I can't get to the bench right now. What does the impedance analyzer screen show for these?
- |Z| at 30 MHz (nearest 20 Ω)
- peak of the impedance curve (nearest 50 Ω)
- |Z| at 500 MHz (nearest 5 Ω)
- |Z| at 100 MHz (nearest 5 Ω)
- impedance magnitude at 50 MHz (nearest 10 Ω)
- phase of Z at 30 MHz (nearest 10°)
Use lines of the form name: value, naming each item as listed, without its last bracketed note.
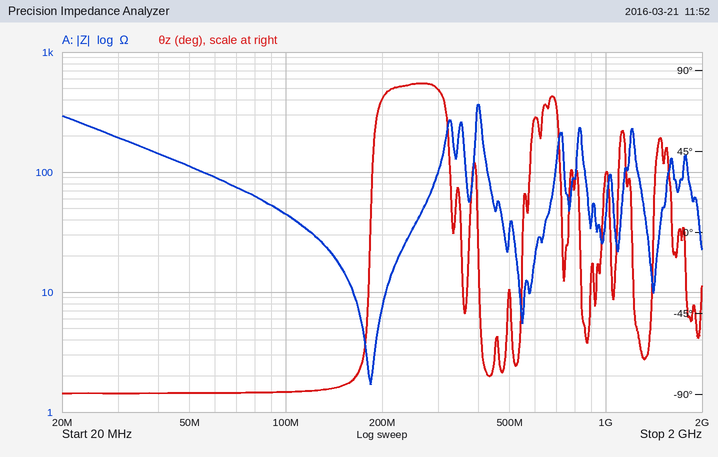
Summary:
|Z| at 30 MHz: 200 Ω
peak of the impedance curve: 350 Ω
|Z| at 500 MHz: 30 Ω
|Z| at 100 MHz: 45 Ω
impedance magnitude at 50 MHz: 110 Ω
phase of Z at 30 MHz: -90°
